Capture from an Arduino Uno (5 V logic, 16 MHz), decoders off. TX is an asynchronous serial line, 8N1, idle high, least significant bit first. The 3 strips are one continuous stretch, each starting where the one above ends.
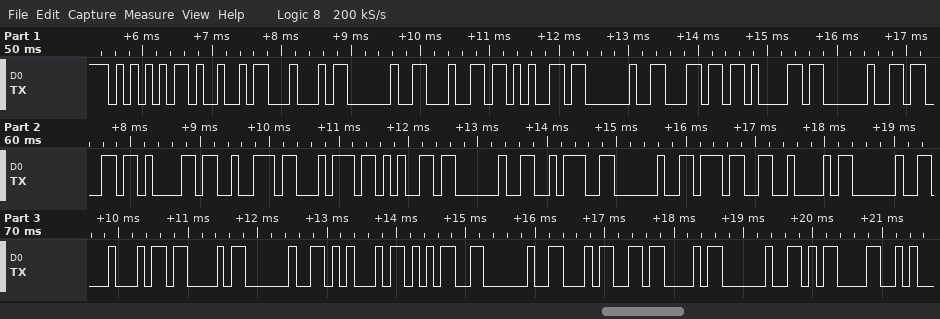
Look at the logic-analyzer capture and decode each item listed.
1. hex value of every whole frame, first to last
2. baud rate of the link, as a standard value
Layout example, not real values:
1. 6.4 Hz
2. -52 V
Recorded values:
1. 55 49 44 20 64 65 20 6C 61 20 63 61 72 74 65 20 3A 20 37 42 20 44 43 20 45 35 20 34 43 20 0D
2. 9600 baud
